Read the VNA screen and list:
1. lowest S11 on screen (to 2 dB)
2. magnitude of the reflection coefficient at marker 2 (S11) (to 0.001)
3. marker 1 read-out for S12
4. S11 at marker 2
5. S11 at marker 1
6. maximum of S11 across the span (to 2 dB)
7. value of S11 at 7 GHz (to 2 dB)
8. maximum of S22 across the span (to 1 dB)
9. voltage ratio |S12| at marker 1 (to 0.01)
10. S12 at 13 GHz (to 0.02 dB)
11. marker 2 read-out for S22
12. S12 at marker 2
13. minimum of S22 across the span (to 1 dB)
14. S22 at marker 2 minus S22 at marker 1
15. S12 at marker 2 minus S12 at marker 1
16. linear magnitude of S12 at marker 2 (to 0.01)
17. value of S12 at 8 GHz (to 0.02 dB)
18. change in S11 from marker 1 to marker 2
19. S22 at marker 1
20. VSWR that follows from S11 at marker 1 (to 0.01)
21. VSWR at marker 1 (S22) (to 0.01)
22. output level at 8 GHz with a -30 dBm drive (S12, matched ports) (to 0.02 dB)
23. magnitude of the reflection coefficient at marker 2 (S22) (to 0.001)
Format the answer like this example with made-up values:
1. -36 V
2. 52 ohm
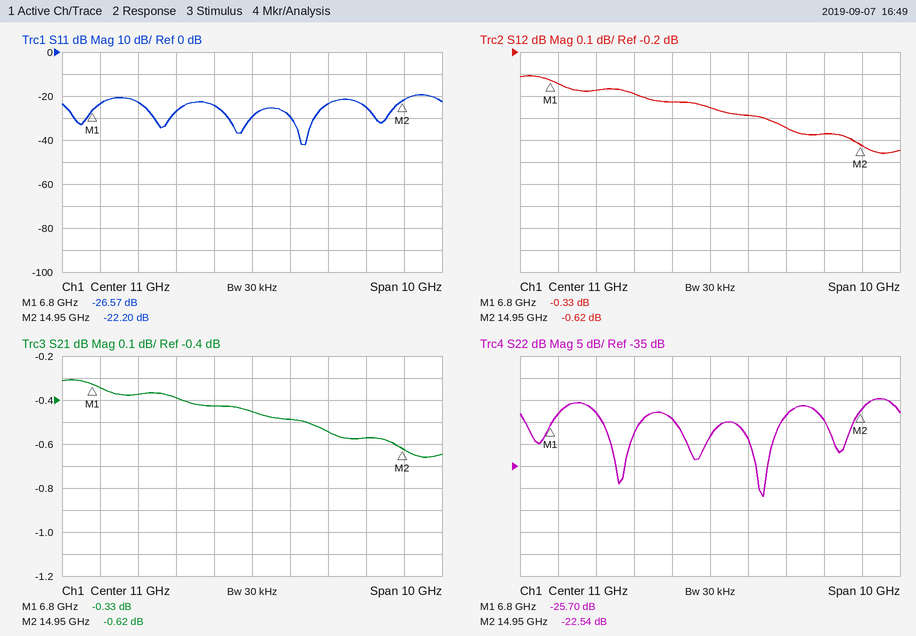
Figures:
1. -42 dB
2. 0.078
3. -0.33 dB
4. -22.20 dB
5. -26.57 dB
6. -20 dB
7. -24 dB
8. -20 dB
9. 0.96
10. -0.54 dB
11. -22.54 dB
12. -0.62 dB
13. -42 dB
14. 3.16 dB
15. -0.29 dB
16. 0.93
17. -0.38 dB
18. 4.37 dB
19. -25.70 dB
20. 1.10
21. 1.11
22. -30.38 dBm
23. 0.075
